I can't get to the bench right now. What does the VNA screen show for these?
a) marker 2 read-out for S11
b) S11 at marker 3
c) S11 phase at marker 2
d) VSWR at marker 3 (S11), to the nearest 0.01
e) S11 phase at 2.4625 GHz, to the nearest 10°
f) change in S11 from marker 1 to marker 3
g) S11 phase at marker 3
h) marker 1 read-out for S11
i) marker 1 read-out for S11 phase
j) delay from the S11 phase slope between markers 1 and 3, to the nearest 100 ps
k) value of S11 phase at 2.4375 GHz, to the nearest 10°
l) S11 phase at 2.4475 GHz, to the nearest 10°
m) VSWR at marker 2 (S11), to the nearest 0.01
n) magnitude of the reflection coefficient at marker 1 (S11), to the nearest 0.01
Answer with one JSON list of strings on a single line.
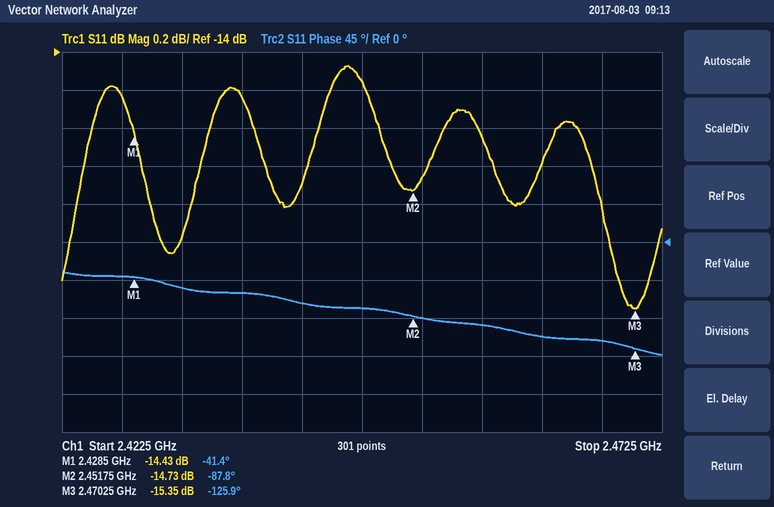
["-14.73 dB", "-15.35 dB", "-87.8°", "1.41", "-110°", "-0.92 dB", "-125.9°", "-14.43 dB", "-41.4°", "5.6 ns", "-60°", "-80°", "1.45", "0.19"]
